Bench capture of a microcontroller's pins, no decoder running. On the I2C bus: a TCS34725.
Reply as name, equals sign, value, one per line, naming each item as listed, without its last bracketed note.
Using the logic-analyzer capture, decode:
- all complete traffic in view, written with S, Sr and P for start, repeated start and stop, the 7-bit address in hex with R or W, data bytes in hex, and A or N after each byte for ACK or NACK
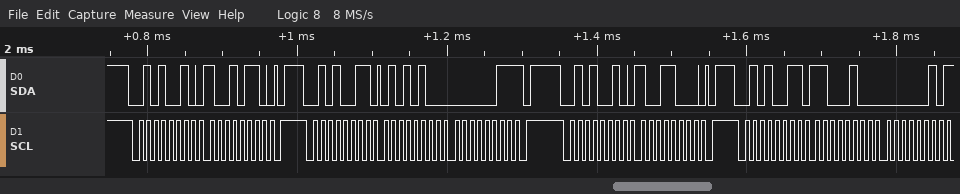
all complete traffic in view, written with S, Sr and P for start, repeated start and stop, the 7-bit address in hex with R or W, data bytes in hex, and A or N after each byte for ACK or NACK = S 29W A 96 A P S 29R A 54 A 03 N P S 29W A 98 A P S 29R A C4 A 02 N
